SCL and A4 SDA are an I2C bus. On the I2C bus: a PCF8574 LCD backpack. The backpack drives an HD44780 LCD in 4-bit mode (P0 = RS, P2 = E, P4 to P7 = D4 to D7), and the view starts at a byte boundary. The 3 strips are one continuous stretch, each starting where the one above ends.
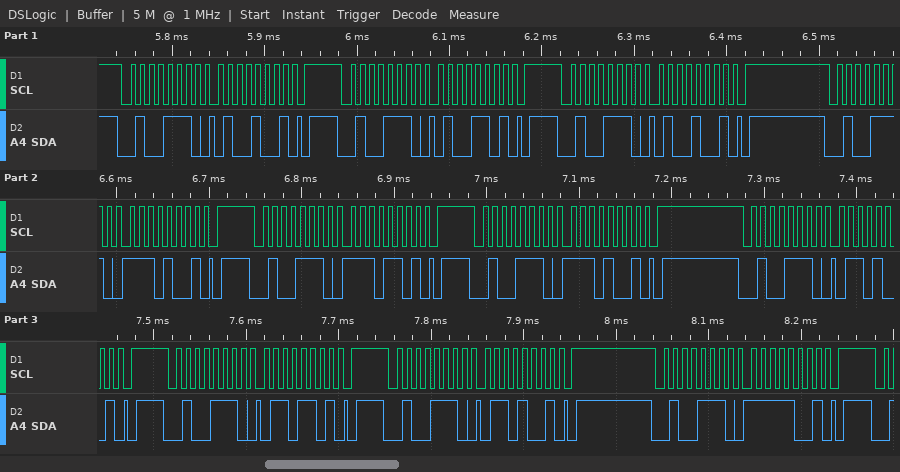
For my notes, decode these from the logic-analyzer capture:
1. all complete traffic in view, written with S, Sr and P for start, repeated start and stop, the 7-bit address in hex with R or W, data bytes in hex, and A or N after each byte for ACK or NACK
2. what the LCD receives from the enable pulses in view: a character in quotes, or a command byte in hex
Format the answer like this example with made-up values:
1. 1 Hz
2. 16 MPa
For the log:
1. S 27W A 49 A P S 27W A 4D A P S 27W A 49 A P S 27W A E9 A P S 27W A ED A P S 27W A E9 A P S 27W A 69 A P S 27W A 6D A P S 27W A 69 A P S 27W A F9 A P
2. 'N'
